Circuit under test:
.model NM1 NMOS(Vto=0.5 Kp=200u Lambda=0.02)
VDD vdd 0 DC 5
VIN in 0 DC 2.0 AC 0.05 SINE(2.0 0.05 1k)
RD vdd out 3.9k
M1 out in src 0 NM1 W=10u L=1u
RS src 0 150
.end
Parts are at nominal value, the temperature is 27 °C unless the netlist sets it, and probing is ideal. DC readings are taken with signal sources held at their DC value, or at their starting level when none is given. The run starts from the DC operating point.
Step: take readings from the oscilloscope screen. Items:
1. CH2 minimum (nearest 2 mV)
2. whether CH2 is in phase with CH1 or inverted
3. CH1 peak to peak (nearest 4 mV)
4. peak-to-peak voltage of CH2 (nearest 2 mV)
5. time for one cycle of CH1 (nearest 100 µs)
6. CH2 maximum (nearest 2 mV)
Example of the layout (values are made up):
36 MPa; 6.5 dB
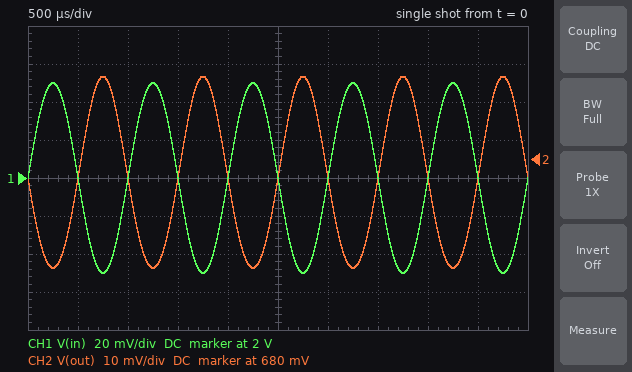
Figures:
652 mV; inverted; 100 mV; 50 mV; 1.0 ms; 702 mV
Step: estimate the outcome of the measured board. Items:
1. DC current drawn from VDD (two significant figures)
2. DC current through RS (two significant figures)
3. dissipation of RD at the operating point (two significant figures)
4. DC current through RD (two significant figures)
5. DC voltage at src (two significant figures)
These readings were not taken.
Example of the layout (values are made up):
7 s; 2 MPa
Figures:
1.1 mA; 1.1 mA; 4.8 mW; 1.1 mA; 170 mV
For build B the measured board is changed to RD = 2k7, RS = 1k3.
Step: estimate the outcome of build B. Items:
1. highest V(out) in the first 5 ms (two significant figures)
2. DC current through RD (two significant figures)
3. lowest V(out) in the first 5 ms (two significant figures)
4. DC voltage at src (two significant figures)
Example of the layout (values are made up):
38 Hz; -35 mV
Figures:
3.5 V; 580 µA; 3.4 V; 760 mV
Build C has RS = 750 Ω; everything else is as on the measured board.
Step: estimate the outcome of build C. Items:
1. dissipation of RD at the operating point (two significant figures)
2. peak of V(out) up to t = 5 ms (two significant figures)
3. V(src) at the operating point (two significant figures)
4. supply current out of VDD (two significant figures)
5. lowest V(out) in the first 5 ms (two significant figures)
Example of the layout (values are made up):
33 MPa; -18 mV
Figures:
2.6 mW; 2.0 V; 610 mV; 810 µA; 1.7 V
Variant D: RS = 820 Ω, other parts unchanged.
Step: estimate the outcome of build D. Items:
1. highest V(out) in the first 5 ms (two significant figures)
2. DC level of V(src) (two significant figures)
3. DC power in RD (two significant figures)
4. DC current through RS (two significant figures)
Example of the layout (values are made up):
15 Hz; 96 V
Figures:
2.1 V; 630 mV; 2.3 mW; 770 µA
